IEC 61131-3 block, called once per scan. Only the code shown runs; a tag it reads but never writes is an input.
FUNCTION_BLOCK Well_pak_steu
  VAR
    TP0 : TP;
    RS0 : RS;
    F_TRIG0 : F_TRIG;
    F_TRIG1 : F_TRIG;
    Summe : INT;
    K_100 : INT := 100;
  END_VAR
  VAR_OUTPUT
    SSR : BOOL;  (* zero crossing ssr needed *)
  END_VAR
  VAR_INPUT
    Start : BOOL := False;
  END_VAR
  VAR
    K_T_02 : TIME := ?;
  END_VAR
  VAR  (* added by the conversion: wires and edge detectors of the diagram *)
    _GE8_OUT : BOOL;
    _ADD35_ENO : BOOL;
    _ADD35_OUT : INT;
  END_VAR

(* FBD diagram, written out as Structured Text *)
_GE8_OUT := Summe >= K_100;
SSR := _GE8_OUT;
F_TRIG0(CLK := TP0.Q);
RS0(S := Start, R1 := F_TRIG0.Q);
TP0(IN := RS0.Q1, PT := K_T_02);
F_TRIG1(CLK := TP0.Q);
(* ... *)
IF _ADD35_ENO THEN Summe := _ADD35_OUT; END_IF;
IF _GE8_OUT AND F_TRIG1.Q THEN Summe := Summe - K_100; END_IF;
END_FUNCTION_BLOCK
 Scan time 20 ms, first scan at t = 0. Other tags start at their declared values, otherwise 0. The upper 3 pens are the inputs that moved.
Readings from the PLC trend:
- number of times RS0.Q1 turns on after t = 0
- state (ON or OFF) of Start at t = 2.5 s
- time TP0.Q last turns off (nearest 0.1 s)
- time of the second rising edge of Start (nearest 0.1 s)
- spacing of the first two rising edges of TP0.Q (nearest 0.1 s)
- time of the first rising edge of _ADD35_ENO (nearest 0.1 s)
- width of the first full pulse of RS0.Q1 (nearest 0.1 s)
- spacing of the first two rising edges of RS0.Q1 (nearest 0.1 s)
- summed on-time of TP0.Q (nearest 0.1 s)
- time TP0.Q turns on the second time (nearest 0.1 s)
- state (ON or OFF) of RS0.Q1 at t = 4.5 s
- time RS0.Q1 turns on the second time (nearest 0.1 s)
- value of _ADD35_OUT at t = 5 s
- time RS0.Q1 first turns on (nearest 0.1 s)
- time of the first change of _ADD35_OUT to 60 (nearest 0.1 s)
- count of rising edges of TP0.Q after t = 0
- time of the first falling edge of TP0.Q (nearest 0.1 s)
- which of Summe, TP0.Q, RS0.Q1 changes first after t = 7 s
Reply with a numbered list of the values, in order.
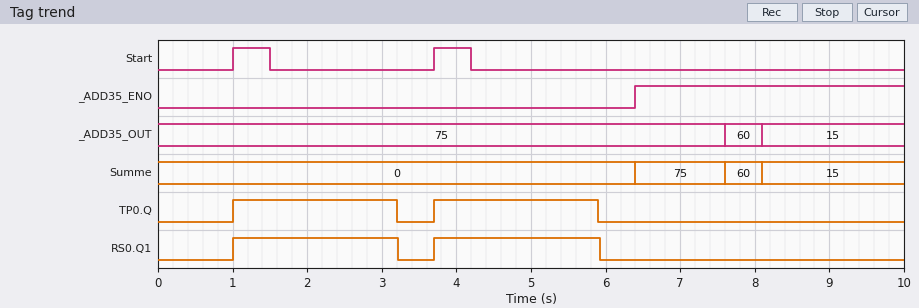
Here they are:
1. 2
2. OFF
3. 5.9 s
4. 3.7 s
5. 2.7 s
6. 6.4 s
7. 2.2 s
8. 2.7 s
9. 4.4 s
10. 3.7 s
11. ON
12. 3.7 s
13. 75
14. 1.0 s
15. 7.6 s
16. 2
17. 3.2 s
18. Summe
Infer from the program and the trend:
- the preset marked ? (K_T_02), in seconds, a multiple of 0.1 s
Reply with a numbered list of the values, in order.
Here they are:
1. 2.2 s
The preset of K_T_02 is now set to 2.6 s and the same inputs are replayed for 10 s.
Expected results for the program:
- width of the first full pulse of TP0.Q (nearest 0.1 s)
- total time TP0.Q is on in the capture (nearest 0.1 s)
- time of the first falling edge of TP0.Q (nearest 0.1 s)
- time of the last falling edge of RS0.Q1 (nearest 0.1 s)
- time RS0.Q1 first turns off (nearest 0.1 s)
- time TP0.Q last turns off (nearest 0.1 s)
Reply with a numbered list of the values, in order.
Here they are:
1. 2.6 s
2. 5.2 s
3. 3.6 s
4. 6.3 s
5. 3.6 s
6. 6.3 s
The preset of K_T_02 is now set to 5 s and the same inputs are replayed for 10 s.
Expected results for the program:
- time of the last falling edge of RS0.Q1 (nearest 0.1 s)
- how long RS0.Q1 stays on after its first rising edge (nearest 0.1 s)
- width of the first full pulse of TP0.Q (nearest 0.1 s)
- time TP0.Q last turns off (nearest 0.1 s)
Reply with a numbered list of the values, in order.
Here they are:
1. 6.0 s
2. 5.0 s
3. 5.0 s
4. 6.0 s
